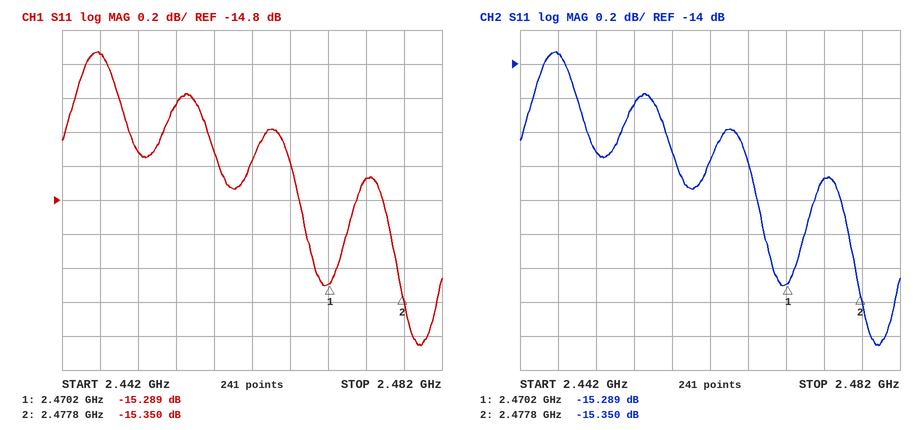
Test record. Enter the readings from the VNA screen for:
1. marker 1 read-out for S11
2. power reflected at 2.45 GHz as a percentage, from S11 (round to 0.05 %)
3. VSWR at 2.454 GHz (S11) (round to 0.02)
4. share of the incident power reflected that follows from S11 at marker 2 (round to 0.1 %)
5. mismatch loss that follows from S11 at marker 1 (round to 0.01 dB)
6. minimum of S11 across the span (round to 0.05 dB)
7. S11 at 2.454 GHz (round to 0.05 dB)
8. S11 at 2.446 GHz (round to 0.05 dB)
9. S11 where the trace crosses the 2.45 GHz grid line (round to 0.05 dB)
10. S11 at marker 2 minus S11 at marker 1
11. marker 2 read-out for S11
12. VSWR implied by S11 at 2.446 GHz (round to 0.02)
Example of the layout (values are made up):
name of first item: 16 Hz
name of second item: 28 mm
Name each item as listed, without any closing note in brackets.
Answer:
marker 1 read-out for S11: -15.289 dB
power reflected at 2.45 GHz as a percentage, from S11: 3.55 %
VSWR at 2.454 GHz (S11): 1.48
share of the incident power reflected that follows from S11 at marker 2: 2.9 %
mismatch loss that follows from S11 at marker 1: 0.13 dB
minimum of S11 across the span: -15.65 dB
S11 at 2.454 GHz: -14.25 dB
S11 at 2.446 GHz: -13.95 dB
S11 where the trace crosses the 2.45 GHz grid line: -14.50 dB
S11 at marker 2 minus S11 at marker 1: -0.061 dB
marker 2 read-out for S11: -15.350 dB
VSWR implied by S11 at 2.446 GHz: 1.50
